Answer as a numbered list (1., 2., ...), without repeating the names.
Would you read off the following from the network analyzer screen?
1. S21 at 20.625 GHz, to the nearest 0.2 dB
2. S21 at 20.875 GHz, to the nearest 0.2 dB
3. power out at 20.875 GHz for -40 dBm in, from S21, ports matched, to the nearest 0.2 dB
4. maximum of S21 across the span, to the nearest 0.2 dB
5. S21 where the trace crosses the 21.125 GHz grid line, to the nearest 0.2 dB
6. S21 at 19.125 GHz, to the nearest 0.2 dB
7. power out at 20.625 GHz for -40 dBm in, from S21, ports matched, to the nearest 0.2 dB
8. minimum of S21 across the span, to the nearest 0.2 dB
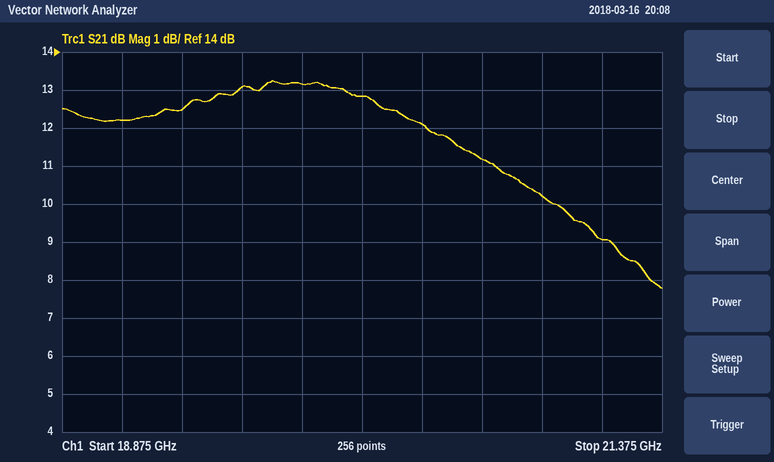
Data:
1. 11.2 dB
2. 10.2 dB
3. -29.8 dBm
4. 13.2 dB
5. 9.0 dB
6. 12.2 dB
7. -28.8 dBm
8. 7.8 dB
